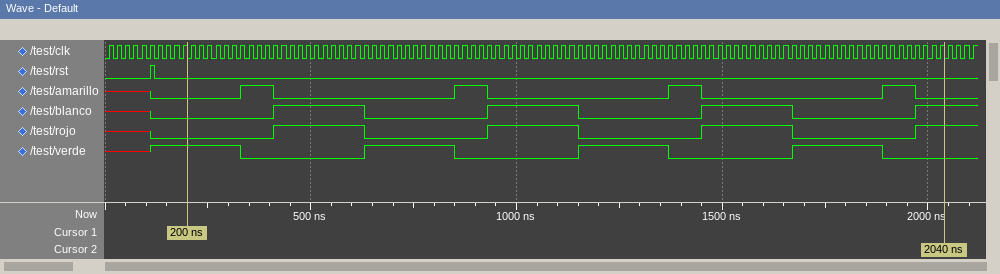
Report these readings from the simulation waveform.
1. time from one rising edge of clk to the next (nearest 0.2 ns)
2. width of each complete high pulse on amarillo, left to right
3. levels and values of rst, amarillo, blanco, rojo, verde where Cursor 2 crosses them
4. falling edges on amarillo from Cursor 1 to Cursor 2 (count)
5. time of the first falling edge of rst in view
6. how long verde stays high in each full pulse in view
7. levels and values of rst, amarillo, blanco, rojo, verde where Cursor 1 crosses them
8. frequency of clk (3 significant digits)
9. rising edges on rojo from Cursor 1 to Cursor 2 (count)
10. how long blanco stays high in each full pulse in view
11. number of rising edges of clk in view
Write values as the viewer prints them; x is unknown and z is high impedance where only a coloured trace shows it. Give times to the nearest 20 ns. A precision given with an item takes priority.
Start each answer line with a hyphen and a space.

- 20 ns
- 80 ns, 80 ns, 80 ns, 80 ns
- rst=0, amarillo=0, blanco=1, rojo=1, verde=0
- 4
- 120 ns
- 220 ns, 220 ns, 220 ns
- rst=0, amarillo=0, blanco=0, rojo=0, verde=1
- 50.0 MHz
- 4
- 220 ns, 220 ns, 220 ns
- 106
